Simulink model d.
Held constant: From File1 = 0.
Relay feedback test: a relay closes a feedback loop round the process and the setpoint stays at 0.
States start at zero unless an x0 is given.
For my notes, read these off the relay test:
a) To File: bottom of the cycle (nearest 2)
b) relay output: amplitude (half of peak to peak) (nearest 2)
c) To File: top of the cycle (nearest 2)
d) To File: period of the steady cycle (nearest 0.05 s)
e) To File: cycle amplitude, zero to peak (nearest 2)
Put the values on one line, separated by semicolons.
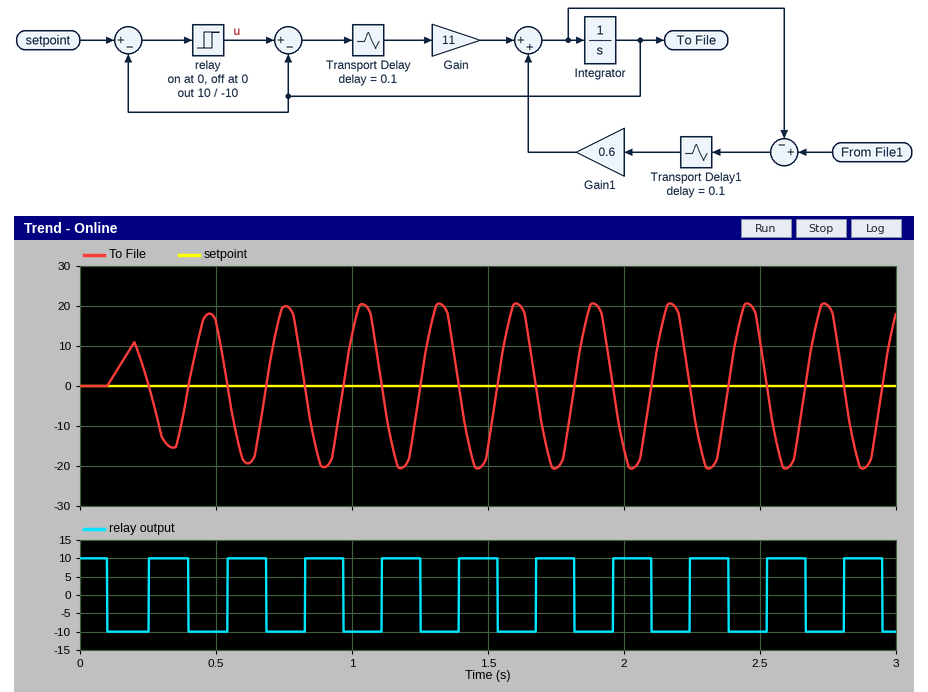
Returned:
-20; 10; 20; 0.30 s; 20
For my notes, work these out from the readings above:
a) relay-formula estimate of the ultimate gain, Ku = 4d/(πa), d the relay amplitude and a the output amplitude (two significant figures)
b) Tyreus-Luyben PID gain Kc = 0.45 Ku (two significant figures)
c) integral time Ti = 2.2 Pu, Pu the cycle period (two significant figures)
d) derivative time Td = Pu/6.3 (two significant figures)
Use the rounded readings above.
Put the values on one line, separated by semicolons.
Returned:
0.64; 0.29; 0.66 s; 0.048 s
